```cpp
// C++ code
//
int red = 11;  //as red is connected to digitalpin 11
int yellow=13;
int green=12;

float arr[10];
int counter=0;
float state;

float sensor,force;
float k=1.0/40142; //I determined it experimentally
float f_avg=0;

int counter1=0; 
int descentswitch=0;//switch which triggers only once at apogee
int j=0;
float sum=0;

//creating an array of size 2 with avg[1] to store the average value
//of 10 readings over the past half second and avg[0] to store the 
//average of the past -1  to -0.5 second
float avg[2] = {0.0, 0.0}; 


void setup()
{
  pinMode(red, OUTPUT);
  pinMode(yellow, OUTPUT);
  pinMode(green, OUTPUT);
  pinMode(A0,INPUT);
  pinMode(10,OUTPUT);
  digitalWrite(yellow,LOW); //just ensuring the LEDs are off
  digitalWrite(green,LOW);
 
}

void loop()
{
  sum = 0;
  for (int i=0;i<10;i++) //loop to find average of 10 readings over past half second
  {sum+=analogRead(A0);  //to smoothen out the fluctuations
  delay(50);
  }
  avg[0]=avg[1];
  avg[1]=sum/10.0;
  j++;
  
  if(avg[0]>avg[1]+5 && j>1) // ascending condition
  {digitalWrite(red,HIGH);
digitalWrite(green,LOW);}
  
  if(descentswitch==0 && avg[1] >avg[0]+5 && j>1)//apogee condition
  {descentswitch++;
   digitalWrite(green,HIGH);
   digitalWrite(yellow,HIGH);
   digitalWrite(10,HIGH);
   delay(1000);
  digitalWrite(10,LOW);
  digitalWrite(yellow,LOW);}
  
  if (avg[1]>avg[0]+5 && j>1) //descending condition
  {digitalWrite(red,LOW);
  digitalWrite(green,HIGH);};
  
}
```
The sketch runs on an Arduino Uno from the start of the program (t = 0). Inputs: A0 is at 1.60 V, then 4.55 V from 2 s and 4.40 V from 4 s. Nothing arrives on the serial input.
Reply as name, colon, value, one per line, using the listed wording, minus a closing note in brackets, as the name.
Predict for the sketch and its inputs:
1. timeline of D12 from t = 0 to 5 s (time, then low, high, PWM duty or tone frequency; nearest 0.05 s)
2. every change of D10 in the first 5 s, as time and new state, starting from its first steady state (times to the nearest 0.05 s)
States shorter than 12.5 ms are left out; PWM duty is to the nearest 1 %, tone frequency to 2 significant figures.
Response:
timeline of D12 from t = 0 to 5 s: 0 s low; 2.5 s high; 4.5 s low
every change of D10 in the first 5 s, as time and new state, starting from its first steady state: 0 s low; 2.5 s high; 3.5 s low
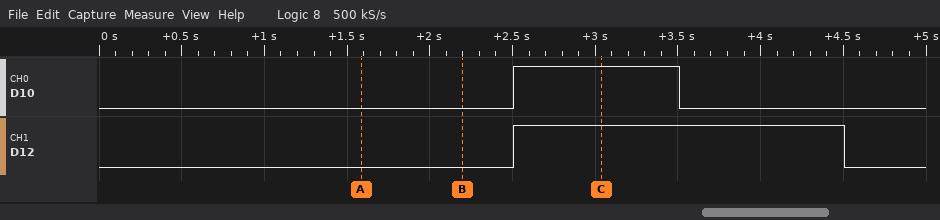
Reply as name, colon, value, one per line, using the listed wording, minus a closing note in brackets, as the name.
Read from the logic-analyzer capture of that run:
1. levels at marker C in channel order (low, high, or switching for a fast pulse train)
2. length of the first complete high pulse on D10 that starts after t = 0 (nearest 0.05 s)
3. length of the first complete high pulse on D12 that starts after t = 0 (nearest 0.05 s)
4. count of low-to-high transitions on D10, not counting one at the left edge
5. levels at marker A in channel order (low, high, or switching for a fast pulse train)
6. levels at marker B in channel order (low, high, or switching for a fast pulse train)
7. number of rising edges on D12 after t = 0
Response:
levels at marker C in channel order: D10 high, D12 high
length of the first complete high pulse on D10 that starts after t = 0: 1.00 s
length of the first complete high pulse on D12 that starts after t = 0: 2.00 s
count of low-to-high transitions on D10, not counting one at the left edge: 1
levels at marker A in channel order: D10 low, D12 low
levels at marker B in channel order: D10 low, D12 low
number of rising edges on D12 after t = 0: 1
